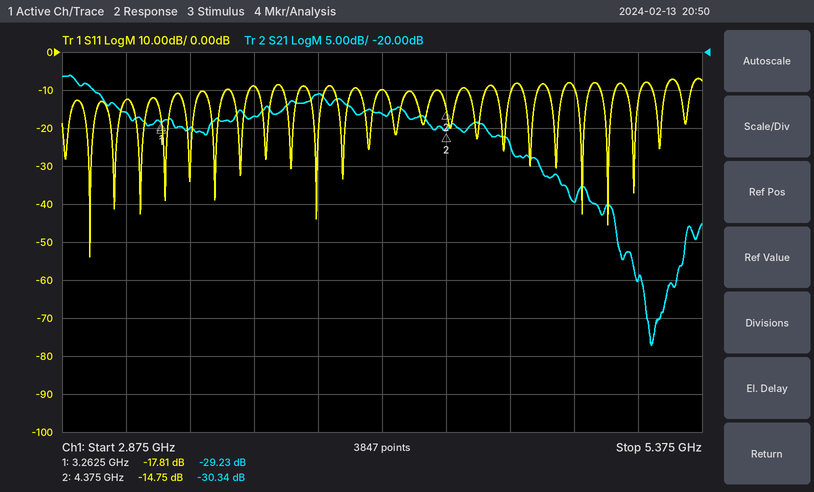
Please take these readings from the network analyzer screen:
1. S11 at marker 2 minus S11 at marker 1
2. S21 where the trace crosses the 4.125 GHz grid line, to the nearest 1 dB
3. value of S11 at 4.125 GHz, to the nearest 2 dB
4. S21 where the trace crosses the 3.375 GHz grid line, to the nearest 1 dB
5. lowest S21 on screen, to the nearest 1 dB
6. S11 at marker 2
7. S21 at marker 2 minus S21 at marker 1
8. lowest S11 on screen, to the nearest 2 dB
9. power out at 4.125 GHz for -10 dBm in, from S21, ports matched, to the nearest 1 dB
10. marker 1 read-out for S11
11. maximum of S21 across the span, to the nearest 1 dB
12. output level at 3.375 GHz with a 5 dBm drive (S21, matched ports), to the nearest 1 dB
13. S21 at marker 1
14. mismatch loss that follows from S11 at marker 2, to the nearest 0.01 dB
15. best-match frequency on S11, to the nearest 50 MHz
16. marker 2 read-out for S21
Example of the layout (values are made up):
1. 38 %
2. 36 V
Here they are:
1. 3.06 dB
2. -28 dB
3. -10 dB
4. -30 dB
5. -59 dB
6. -14.75 dB
7. -1.11 dB
8. -54 dB
9. -38 dBm
10. -17.81 dB
11. -23 dB
12. -25 dBm
13. -29.23 dB
14. 0.15 dB
15. 3.00 GHz
16. -30.34 dB
